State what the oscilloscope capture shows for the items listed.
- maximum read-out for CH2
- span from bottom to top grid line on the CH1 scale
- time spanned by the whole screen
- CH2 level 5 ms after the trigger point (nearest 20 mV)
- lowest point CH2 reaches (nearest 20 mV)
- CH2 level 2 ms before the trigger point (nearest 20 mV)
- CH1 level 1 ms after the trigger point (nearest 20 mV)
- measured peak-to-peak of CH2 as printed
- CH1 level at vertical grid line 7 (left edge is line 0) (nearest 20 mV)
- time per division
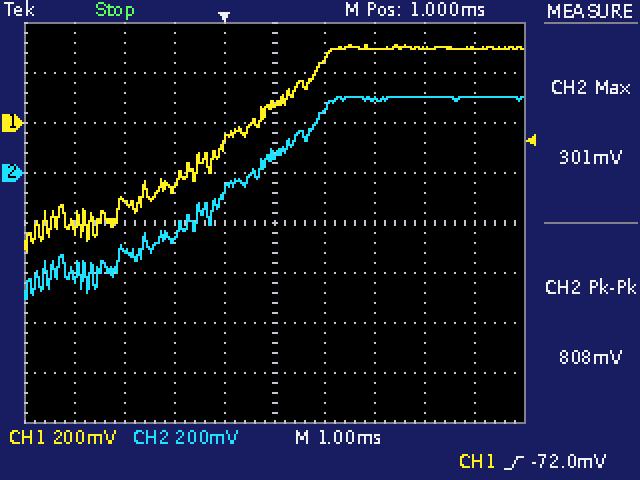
301 mV
1.6 V
10 ms
300 mV
-500 mV
-300 mV
80 mV
808 mV
300 mV
1 ms
